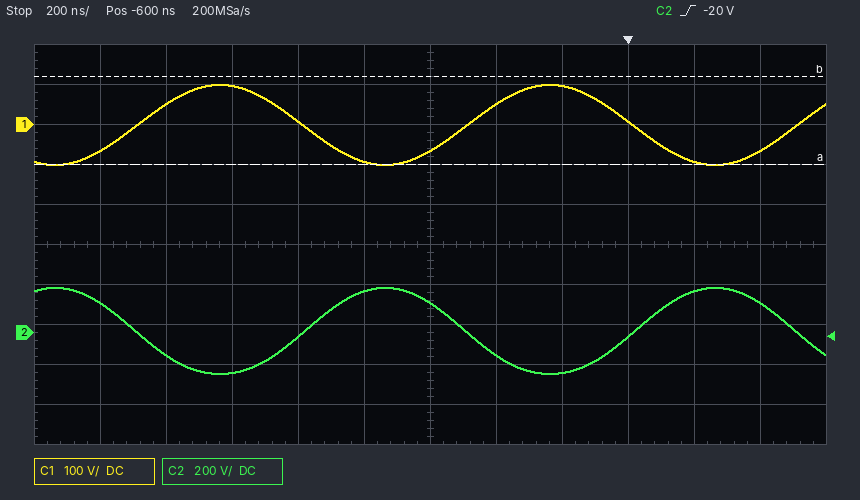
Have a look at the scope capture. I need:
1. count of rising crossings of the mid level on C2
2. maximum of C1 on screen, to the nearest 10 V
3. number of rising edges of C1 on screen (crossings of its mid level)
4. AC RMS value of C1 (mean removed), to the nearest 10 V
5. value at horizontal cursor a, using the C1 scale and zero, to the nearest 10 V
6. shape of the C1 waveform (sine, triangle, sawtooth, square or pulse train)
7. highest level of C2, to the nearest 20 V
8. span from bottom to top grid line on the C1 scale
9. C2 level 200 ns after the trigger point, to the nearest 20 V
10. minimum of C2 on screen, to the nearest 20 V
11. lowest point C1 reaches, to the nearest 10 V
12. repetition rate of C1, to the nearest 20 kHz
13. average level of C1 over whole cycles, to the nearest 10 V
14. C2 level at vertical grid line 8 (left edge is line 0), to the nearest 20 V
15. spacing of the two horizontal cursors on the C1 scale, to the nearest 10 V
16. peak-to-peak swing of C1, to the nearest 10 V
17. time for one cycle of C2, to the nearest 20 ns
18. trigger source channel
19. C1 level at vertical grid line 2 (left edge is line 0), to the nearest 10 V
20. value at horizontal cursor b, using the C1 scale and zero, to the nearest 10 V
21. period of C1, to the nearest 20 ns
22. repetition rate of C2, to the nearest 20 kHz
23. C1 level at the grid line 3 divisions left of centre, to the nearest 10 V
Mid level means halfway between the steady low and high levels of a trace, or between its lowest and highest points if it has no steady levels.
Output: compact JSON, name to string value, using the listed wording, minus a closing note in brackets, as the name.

{"count of rising crossings of the mid level on C2": "2", "maximum of C1 on screen, to the nearest 10 V": "100 V", "number of rising edges of C1 on screen": "3", "AC RMS value of C1 (mean removed), to the nearest 10 V": "70 V", "value at horizontal cursor a, using the C1 scale and zero, to the nearest 10 V": "-100 V", "shape of the C1 waveform": "sine", "highest level of C2, to the nearest 20 V": "220 V", "span from bottom to top grid line on the C1 scale": "1 kV", "C2 level 200 ns after the trigger point, to the nearest 20 V": "200 V", "minimum of C2 on screen, to the nearest 20 V": "-200 V", "lowest point C1 reaches, to the nearest 10 V": "-100 V", "repetition rate of C1, to the nearest 20 kHz": "1.00 MHz", "average level of C1 over whole cycles, to the nearest 10 V": "0 V", "C2 level at vertical grid line 8 (left edge is line 0), to the nearest 20 V": "-200 V", "spacing of the two horizontal cursors on the C1 scale, to the nearest 10 V": "220 V", "peak-to-peak swing of C1, to the nearest 10 V": "200 V", "time for one cycle of C2, to the nearest 20 ns": "1.00 µs", "trigger source channel": "C2", "C1 level at vertical grid line 2 (left edge is line 0), to the nearest 10 V": "50 V", "value at horizontal cursor b, using the C1 scale and zero, to the nearest 10 V": "120 V", "period of C1, to the nearest 20 ns": "1.00 µs", "repetition rate of C2, to the nearest 20 kHz": "1.00 MHz", "C1 level at the grid line 3 divisions left of centre, to the nearest 10 V": "100 V"}
